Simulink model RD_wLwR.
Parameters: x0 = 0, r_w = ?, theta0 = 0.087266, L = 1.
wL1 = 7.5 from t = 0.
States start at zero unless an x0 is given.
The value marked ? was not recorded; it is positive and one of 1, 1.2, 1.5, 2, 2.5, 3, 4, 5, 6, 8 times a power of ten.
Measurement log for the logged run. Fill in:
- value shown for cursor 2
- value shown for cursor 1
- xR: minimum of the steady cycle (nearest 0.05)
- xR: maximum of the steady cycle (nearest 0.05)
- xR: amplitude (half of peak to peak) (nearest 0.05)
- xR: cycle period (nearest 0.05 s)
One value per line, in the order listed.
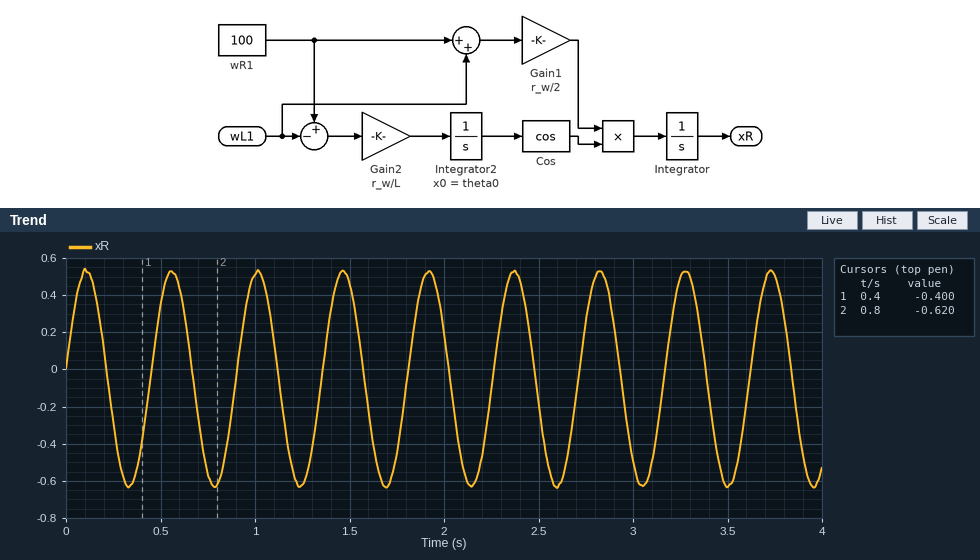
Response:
-0.620
-0.400
-0.65
0.55
0.60
0.45 s
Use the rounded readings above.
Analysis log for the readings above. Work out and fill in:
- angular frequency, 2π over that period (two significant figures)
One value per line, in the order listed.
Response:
14 rad/s
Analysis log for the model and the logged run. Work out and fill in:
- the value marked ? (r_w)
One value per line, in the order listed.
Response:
0.15
